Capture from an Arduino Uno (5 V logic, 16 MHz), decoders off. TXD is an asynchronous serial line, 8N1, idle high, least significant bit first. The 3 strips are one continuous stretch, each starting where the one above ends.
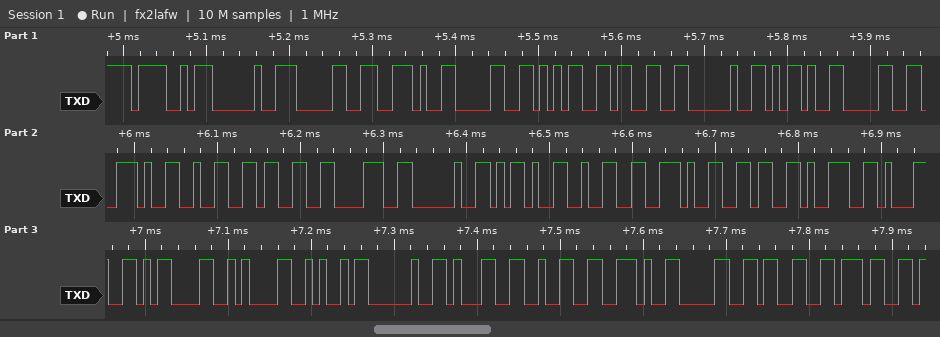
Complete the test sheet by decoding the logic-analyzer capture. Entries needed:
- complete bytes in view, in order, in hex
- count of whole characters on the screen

0x4F 0x20 0x30 0x2E 0x30 0x35 0x33 0x20 0x2D 0x30 0x2E 0x32 0x33 0x38 0x20 0x2D 0x32 0x2E 0x36 0x39 0x31 0x0D 0x0A 0x4A 0x20 0x31 0x32 0x2E 0x30 0x33 0x37
31
